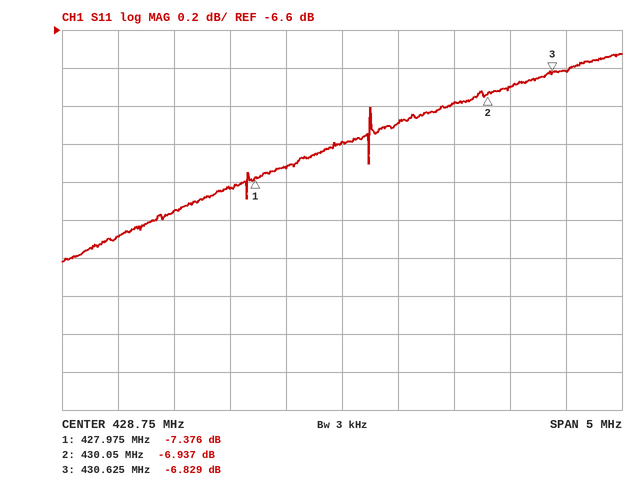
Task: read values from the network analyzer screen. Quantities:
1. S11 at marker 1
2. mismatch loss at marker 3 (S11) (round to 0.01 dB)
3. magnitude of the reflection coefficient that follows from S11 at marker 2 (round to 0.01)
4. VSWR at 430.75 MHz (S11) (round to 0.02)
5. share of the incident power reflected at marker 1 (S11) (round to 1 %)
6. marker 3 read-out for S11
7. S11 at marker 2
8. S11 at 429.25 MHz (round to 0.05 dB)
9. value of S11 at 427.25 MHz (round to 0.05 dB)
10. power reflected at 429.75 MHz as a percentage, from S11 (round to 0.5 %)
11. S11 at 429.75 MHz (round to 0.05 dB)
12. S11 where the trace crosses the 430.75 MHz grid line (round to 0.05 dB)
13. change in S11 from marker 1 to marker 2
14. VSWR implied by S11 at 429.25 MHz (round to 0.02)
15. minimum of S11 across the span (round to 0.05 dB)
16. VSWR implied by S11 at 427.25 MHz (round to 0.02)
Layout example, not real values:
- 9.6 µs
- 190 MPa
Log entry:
- -7.376 dB
- 1.01 dB
- 0.45
- 2.68
- 18 %
- -6.829 dB
- -6.937 dB
- -7.10 dB
- -7.55 dB
- 20.0 %
- -7.00 dB
- -6.80 dB
- 0.439 dB
- 2.58
- -7.80 dB
- 2.44
